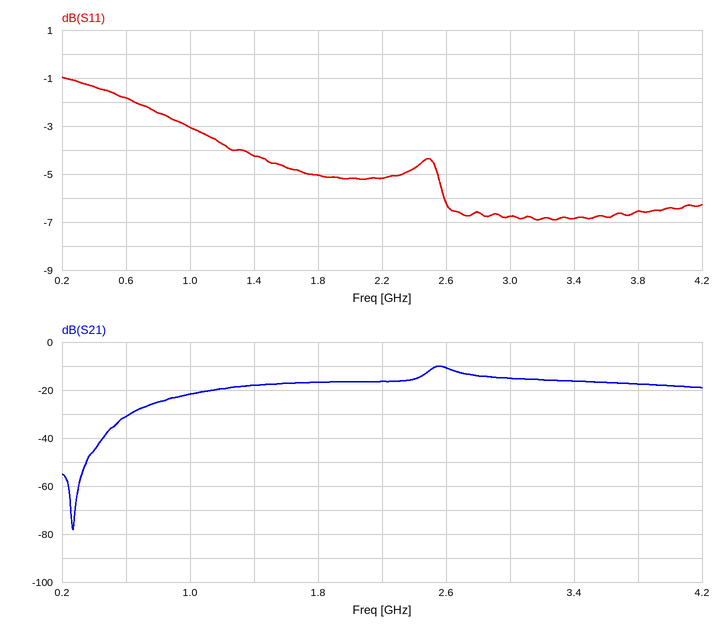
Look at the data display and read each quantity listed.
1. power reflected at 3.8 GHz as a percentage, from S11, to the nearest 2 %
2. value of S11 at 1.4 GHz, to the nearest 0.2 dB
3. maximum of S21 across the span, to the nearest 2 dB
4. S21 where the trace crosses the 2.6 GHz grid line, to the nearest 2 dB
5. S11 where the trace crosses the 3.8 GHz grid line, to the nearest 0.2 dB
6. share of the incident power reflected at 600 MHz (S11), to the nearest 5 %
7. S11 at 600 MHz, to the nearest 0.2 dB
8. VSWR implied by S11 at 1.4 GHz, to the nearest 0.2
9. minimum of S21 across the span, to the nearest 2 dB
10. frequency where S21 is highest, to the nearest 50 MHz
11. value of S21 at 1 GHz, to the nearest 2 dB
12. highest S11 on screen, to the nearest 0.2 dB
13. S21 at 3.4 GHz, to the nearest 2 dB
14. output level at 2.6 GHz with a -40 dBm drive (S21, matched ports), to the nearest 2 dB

22 %
-4.2 dB
-10 dB
-10 dB
-6.6 dB
65 %
-1.8 dB
4.2
-78 dB
2.55 GHz
-22 dB
-1.0 dB
-16 dB
-50 dBm
